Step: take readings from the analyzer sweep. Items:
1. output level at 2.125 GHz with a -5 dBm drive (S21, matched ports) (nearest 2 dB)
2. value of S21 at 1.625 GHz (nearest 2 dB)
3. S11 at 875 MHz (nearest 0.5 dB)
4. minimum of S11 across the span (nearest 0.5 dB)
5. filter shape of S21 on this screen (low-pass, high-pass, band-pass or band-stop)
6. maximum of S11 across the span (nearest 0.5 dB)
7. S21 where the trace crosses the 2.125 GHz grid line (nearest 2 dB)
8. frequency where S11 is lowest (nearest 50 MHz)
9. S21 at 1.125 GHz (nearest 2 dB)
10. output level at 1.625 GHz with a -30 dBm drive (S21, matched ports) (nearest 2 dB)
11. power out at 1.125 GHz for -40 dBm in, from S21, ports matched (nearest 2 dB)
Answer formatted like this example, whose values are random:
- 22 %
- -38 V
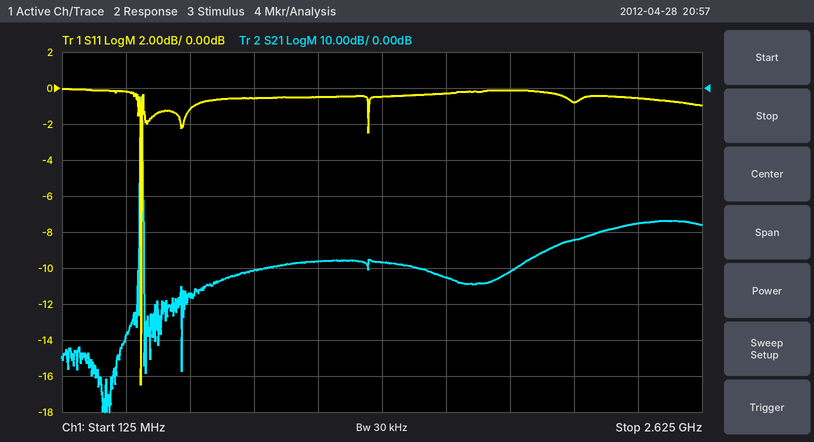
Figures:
- -48 dBm
- -52 dB
- -0.5 dB
- -16.5 dB
- band-pass
- 0.0 dB
- -42 dB
- 450 MHz
- -48 dB
- -82 dBm
- -88 dBm
